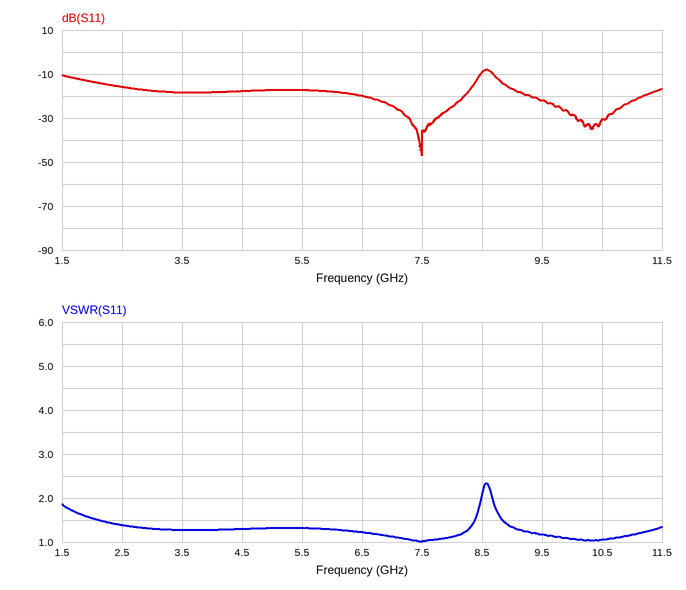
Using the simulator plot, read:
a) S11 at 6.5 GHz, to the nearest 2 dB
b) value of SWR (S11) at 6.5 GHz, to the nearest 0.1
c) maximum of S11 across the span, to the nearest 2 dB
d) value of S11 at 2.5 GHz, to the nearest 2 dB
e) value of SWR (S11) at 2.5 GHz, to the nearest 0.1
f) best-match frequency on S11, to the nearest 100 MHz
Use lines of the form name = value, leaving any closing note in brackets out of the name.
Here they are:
S11 at 6.5 GHz, to the nearest 2 dB = -20 dB
value of SWR (S11) at 6.5 GHz, to the nearest 0.1 = 1.2
maximum of S11 across the span, to the nearest 2 dB = -8 dB
value of S11 at 2.5 GHz, to the nearest 2 dB = -16 dB
value of SWR (S11) at 2.5 GHz, to the nearest 0.1 = 1.4
best-match frequency on S11, to the nearest 100 MHz = 7.5 GHz
